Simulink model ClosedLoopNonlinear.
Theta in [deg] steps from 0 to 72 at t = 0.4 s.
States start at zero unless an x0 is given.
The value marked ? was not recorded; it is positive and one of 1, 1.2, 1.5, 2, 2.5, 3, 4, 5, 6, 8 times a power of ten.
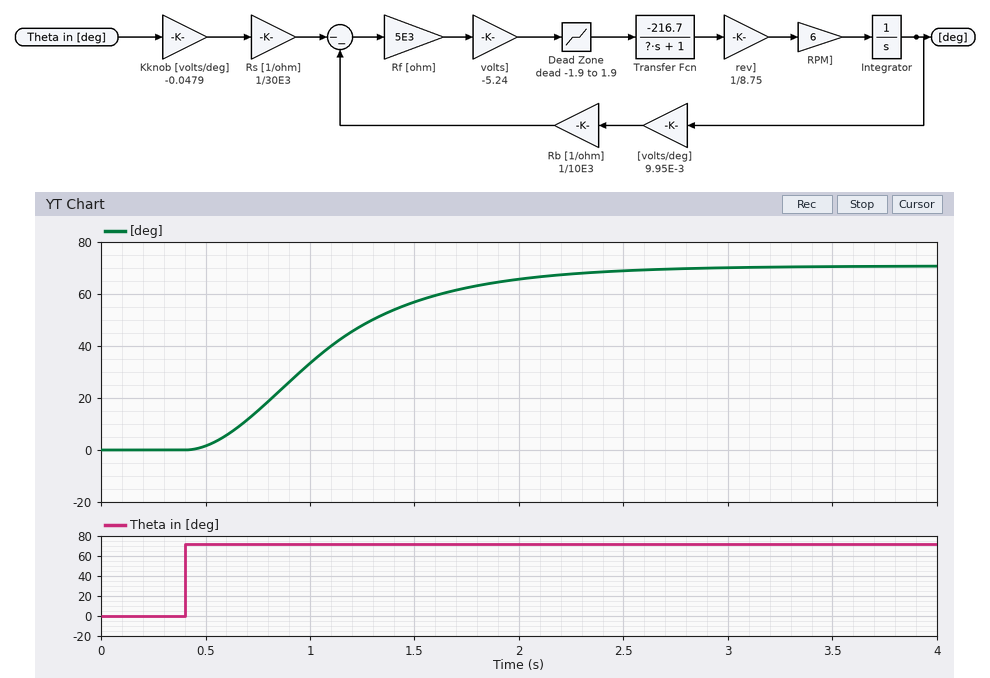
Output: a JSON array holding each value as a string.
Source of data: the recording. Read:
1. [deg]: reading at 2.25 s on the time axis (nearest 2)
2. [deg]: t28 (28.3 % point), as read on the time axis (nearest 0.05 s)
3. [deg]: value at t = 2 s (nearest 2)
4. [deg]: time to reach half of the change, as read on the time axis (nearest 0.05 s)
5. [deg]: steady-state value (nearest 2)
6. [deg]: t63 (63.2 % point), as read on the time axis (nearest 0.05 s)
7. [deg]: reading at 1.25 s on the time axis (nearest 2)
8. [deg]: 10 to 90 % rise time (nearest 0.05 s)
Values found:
["68", "0.80 s", "66", "1.05 s", "70", "1.20 s", "48", "1.20 s"]
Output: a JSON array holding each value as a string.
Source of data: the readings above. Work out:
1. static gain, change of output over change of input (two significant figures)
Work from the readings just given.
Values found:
["0.97"]
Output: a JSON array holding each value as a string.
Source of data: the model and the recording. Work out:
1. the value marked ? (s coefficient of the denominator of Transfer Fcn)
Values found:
["0.5"]
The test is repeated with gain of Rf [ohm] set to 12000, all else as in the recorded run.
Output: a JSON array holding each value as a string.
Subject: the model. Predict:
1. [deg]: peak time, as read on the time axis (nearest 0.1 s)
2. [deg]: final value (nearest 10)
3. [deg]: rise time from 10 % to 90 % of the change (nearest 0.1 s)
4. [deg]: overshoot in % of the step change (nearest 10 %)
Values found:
["1.5 s", "120", "0.4 s", "40 %"]
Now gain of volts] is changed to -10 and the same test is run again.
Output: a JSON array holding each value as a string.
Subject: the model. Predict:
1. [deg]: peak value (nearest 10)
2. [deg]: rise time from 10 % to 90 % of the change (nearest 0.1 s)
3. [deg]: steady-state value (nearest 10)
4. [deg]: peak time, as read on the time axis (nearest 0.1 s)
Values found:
["160", "0.8 s", "150", "2.2 s"]
